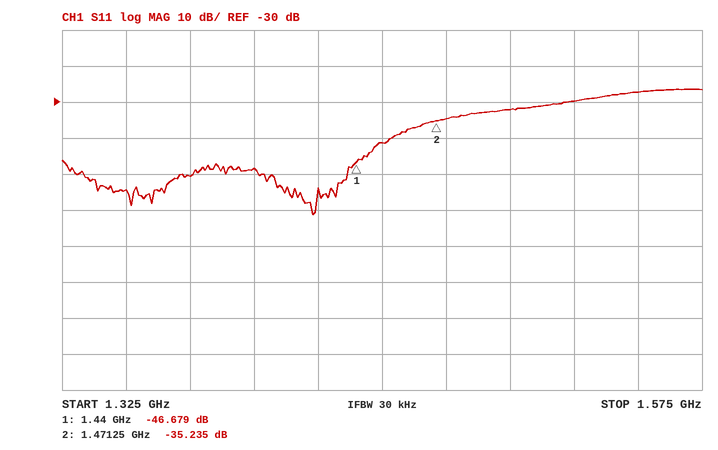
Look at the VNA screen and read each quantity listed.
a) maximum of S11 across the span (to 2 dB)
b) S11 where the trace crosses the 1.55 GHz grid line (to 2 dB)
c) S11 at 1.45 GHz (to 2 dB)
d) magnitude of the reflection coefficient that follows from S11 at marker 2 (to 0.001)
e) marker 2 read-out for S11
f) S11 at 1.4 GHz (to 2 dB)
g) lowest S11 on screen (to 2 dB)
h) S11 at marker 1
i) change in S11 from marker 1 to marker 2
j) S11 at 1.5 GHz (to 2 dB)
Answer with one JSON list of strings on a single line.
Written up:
["-26 dB", "-28 dB", "-42 dB", "0.017", "-35.235 dB", "-48 dB", "-62 dB", "-46.679 dB", "11.444 dB", "-32 dB"]
